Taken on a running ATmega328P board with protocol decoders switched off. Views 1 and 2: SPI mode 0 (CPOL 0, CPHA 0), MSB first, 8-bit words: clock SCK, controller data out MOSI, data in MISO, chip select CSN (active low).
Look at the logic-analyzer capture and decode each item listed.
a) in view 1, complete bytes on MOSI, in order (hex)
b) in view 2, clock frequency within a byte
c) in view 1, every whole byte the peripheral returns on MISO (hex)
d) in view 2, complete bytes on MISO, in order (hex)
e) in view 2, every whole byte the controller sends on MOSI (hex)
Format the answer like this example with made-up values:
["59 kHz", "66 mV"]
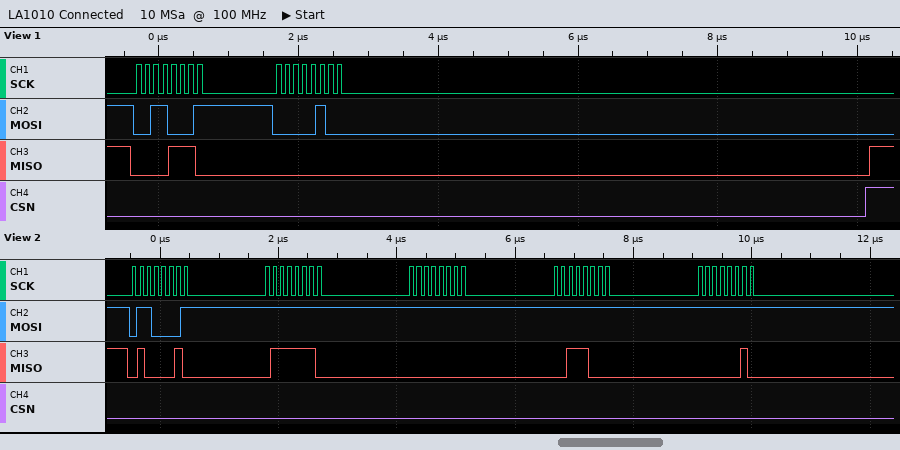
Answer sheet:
["31 04", "8 MHz", "0E 00", "42 7E 00 38 02", "61 FF FF FF FF"]
